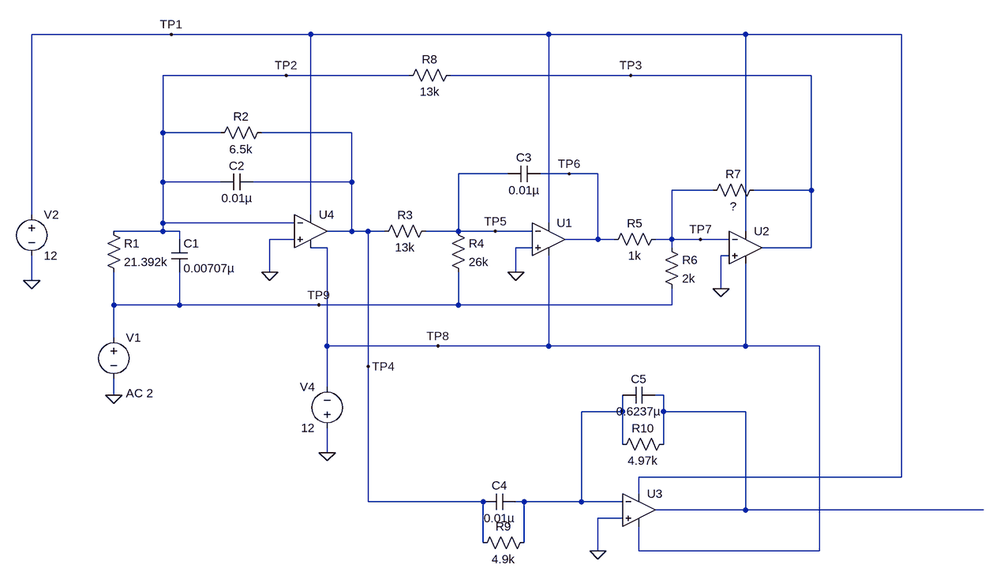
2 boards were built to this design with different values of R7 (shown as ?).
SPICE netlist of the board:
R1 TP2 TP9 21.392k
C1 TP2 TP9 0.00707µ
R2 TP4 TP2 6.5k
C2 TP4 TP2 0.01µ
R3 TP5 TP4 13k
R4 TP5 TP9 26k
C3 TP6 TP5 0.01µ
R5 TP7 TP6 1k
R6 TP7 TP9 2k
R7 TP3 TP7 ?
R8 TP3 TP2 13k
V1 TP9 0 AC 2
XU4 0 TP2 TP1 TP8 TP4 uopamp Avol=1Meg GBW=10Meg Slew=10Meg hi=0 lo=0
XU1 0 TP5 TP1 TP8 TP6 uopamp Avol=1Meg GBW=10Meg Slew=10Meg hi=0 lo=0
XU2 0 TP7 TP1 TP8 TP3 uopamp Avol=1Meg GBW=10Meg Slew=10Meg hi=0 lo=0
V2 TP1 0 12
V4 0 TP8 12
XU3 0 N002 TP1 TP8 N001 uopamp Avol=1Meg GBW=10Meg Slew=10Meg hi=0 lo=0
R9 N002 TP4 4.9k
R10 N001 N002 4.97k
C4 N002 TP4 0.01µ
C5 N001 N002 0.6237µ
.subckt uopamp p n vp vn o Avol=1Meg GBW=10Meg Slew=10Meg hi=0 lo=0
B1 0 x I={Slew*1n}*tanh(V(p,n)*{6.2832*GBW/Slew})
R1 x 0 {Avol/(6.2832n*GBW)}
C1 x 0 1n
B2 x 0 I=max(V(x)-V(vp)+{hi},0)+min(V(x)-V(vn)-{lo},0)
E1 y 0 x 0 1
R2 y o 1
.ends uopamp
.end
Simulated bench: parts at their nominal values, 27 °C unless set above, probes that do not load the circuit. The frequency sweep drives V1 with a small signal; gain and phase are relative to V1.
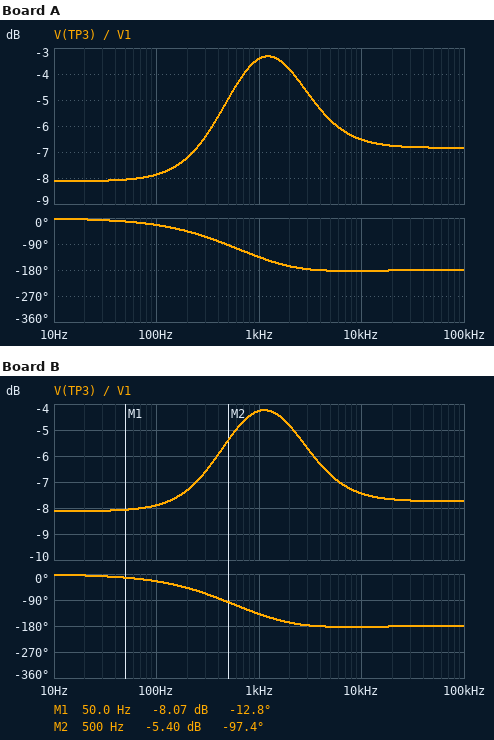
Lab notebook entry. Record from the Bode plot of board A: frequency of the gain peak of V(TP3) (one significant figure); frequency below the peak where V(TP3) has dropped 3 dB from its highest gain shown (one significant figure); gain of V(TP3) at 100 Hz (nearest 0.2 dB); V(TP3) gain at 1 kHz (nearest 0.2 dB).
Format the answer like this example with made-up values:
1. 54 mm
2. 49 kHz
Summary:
1. 1 kHz
2. 300 Hz
3. -7.8 dB
4. -3.4 dB
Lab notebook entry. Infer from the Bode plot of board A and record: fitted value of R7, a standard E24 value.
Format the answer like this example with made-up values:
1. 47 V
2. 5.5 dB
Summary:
1. 910 Ω
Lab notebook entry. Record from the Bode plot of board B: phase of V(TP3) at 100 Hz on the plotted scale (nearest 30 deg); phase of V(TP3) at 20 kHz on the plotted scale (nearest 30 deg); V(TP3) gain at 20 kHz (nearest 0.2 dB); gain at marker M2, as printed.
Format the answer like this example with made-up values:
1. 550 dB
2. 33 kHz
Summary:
1. -30 deg
2. -180 deg
3. -7.6 dB
4. -5.40 dB
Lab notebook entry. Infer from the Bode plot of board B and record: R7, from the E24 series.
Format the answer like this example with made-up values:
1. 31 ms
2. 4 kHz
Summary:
1. 820 Ω
